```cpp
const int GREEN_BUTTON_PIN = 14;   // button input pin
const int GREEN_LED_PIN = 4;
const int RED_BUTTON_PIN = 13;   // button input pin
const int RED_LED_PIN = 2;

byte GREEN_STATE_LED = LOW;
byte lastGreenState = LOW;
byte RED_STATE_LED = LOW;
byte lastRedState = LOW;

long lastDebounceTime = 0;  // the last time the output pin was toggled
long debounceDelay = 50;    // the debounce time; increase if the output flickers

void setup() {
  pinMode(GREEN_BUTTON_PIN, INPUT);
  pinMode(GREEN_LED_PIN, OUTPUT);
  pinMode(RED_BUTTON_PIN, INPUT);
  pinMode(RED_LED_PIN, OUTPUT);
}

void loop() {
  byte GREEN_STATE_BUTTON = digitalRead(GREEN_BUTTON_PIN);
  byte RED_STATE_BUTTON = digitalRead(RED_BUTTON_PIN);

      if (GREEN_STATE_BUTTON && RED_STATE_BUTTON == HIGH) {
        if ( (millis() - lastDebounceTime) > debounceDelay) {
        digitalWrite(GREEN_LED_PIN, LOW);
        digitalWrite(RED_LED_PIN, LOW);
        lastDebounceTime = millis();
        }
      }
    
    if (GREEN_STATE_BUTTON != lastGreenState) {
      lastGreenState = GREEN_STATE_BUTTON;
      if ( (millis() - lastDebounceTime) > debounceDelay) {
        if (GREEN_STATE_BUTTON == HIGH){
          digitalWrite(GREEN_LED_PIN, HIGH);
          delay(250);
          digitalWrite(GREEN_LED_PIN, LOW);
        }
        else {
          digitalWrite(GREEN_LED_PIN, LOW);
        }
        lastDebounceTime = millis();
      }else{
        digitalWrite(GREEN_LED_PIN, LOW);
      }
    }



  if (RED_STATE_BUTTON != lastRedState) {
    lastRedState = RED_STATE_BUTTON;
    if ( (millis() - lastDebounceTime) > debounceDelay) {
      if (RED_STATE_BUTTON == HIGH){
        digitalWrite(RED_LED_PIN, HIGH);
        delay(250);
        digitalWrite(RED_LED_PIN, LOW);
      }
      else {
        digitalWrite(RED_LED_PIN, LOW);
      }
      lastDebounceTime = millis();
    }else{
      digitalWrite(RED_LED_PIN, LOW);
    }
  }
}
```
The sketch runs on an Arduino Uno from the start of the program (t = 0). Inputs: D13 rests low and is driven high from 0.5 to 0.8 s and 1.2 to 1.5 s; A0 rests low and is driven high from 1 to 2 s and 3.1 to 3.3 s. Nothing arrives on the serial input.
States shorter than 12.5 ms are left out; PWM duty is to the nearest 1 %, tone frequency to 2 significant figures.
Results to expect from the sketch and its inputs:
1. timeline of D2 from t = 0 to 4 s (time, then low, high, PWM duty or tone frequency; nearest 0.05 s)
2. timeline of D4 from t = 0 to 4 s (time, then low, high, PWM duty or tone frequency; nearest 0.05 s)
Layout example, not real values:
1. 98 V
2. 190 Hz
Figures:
1. 0 s low; 0.5 s high; 0.75 s low
2. 0 s low; 1 s high; 1.25 s low; 3.1 s high; 3.35 s low
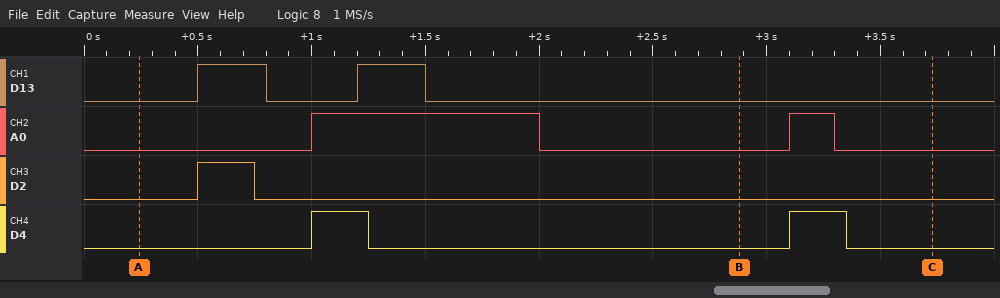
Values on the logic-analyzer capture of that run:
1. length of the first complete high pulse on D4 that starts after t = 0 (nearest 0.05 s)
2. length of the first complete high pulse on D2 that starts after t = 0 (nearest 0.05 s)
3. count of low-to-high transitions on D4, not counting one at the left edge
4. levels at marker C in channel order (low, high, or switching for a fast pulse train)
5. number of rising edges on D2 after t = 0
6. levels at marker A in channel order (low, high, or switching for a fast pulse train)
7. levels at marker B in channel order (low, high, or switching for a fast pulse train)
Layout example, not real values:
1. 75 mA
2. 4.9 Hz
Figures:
1. 0.25 s
2. 0.25 s
3. 2
4. D13 low, A0 low, D2 low, D4 low
5. 1
6. D13 low, A0 low, D2 low, D4 low
7. D13 low, A0 low, D2 low, D4 low
